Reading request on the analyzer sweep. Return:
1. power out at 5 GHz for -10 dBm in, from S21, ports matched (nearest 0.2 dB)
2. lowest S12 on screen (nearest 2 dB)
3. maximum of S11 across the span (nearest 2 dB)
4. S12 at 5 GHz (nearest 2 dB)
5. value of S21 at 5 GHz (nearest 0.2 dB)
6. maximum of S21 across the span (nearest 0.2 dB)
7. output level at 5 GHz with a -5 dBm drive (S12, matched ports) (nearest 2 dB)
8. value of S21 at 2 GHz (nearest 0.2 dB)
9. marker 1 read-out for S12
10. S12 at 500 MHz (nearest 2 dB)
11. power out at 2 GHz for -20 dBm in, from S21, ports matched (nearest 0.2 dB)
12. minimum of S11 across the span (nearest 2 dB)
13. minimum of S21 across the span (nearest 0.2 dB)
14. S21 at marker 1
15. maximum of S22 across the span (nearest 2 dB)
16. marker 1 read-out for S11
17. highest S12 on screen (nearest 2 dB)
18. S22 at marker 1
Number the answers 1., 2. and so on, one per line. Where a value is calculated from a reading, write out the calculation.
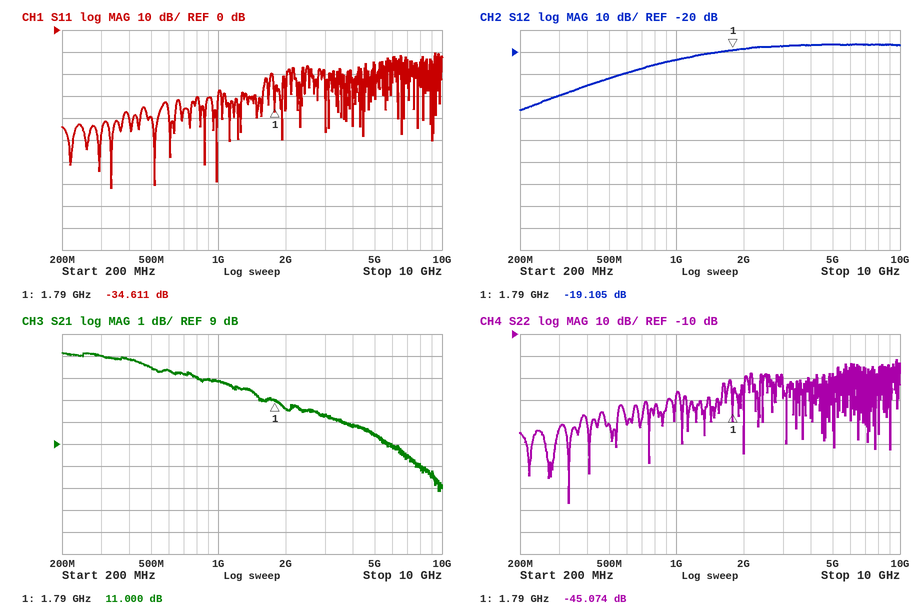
1. -10 dBm + (9.4 dB) = -0.6 dBm
2. -46 dB
3. -10 dB
4. -16 dB
5. 9.4 dB
6. 13.2 dB
7. -5 dBm + (-16 dB) = -22 dBm
8. 10.6 dB
9. -19.105 dB
10. -32 dB
11. -20 dBm + (10.6 dB) = -9.4 dBm
12. -72 dB
13. 6.8 dB
14. 11.000 dB
15. -22 dB
16. -34.611 dB
17. -16 dB
18. -45.074 dB
